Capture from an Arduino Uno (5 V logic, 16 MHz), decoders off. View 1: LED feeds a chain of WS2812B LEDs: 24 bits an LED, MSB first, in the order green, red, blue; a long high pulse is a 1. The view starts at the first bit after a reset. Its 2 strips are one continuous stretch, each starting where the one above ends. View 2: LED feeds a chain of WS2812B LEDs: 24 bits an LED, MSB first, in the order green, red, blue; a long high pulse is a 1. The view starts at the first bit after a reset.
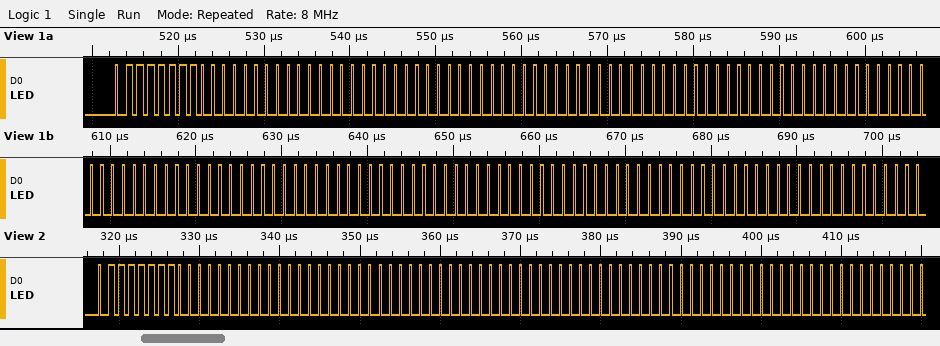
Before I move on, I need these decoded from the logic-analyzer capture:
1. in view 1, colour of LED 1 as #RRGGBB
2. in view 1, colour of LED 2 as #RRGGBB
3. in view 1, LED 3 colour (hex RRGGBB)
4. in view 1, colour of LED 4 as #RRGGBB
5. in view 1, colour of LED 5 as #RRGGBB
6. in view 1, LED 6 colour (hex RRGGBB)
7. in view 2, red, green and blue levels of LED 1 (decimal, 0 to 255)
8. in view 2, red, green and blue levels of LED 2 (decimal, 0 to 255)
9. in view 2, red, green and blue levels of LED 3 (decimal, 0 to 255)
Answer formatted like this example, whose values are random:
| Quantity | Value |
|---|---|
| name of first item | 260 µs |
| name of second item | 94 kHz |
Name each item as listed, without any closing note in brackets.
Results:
| Quantity | Value |
|---|---|
| in view 1, colour of LED 1 as #RRGGBB | #007F00 |
| in view 1, colour of LED 2 as #RRGGBB | #000000 |
| in view 1, LED 3 colour | #000000 |
| in view 1, colour of LED 4 as #RRGGBB | #000000 |
| in view 1, colour of LED 5 as #RRGGBB | #000000 |
| in view 1, LED 6 colour | #000000 |
| in view 2, red, green and blue levels of LED 1 | 0, 127, 0 |
| in view 2, red, green and blue levels of LED 2 | 0, 0, 0 |
| in view 2, red, green and blue levels of LED 3 | 0, 0, 0 |
